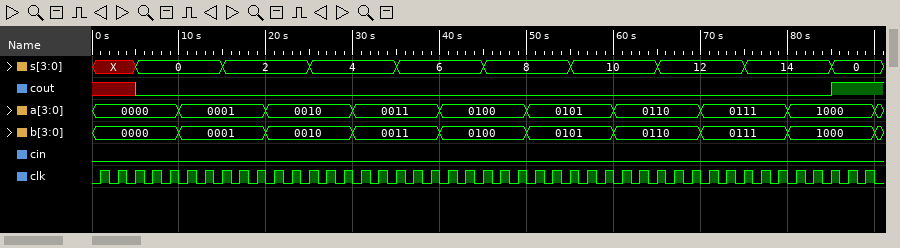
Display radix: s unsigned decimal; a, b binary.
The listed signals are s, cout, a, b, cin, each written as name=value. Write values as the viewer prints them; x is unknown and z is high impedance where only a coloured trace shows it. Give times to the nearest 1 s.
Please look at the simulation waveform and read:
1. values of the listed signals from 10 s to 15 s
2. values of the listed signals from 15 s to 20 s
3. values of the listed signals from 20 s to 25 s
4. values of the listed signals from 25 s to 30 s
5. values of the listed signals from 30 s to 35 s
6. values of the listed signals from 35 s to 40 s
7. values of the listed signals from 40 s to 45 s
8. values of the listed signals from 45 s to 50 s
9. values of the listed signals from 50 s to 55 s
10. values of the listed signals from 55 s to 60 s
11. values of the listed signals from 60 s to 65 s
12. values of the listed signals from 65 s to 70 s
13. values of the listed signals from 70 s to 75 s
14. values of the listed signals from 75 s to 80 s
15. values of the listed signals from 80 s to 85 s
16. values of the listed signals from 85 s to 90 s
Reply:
s=0, cout=0, a=0001, b=0001, cin=0
s=2, cout=0, a=0001, b=0001, cin=0
s=2, cout=0, a=0010, b=0010, cin=0
s=4, cout=0, a=0010, b=0010, cin=0
s=4, cout=0, a=0011, b=0011, cin=0
s=6, cout=0, a=0011, b=0011, cin=0
s=6, cout=0, a=0100, b=0100, cin=0
s=8, cout=0, a=0100, b=0100, cin=0
s=8, cout=0, a=0101, b=0101, cin=0
s=10, cout=0, a=0101, b=0101, cin=0
s=10, cout=0, a=0110, b=0110, cin=0
s=12, cout=0, a=0110, b=0110, cin=0
s=12, cout=0, a=0111, b=0111, cin=0
s=14, cout=0, a=0111, b=0111, cin=0
s=14, cout=0, a=1000, b=1000, cin=0
s=0, cout=1, a=1000, b=1000, cin=0
